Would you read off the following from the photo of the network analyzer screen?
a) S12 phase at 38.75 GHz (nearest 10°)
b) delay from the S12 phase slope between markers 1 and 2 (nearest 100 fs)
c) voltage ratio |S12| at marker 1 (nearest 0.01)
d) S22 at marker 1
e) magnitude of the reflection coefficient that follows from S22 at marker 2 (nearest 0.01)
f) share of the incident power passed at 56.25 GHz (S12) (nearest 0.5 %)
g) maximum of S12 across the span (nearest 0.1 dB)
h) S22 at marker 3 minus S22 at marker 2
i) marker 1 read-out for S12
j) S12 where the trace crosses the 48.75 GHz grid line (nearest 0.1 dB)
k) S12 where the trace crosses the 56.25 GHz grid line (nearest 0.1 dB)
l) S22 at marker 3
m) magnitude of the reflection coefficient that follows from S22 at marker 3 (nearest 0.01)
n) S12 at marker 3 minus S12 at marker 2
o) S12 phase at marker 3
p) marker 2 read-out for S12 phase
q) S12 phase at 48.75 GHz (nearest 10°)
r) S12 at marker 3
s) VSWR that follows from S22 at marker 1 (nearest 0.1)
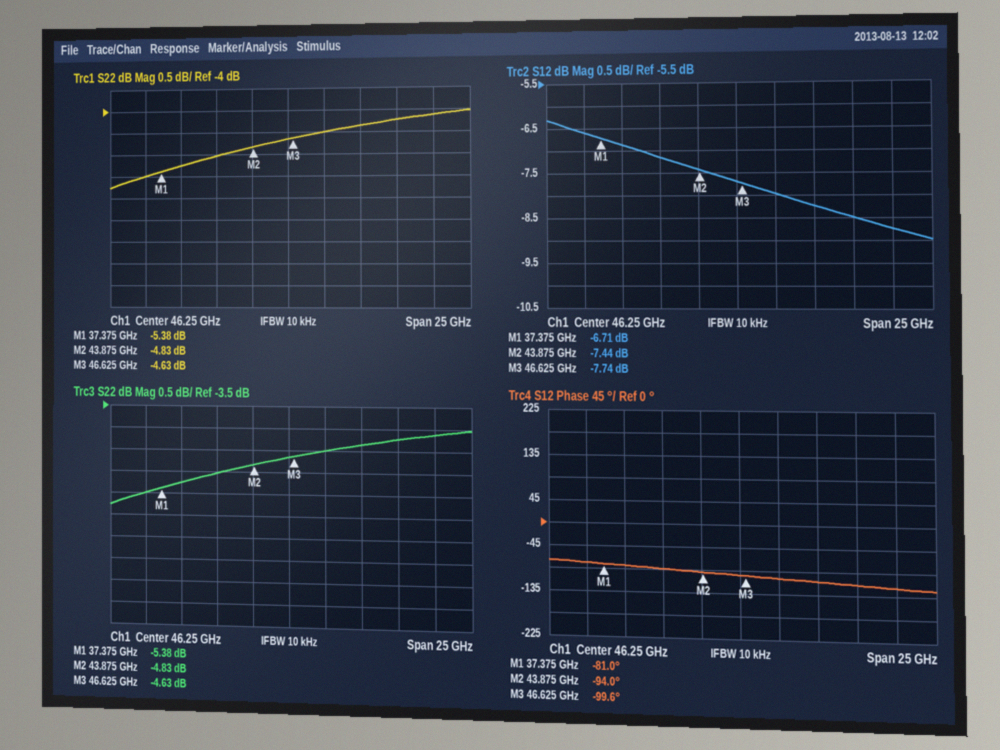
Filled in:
-80°
5.6 ps
0.46
-5.38 dB
0.57
13.5 %
-6.3 dB
0.20 dB
-6.71 dB
-8.0 dB
-8.7 dB
-4.63 dB
0.59
-0.30 dB
-99.6°
-94.0°
-100°
-7.74 dB
3.3
